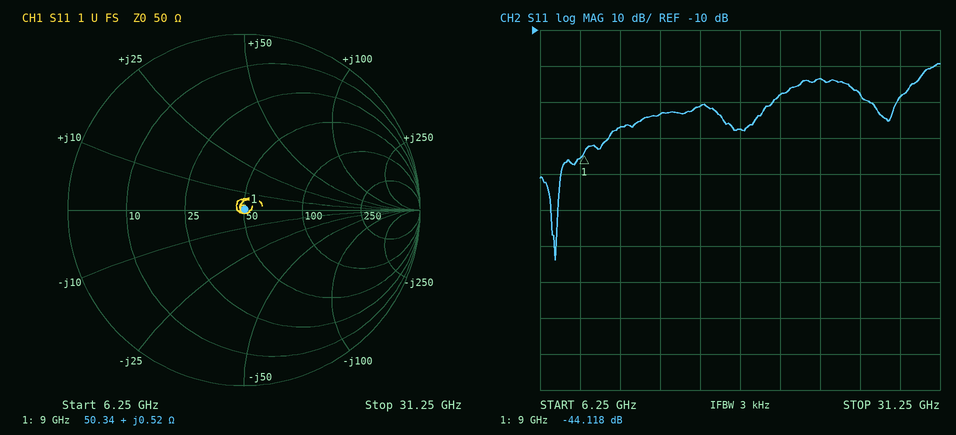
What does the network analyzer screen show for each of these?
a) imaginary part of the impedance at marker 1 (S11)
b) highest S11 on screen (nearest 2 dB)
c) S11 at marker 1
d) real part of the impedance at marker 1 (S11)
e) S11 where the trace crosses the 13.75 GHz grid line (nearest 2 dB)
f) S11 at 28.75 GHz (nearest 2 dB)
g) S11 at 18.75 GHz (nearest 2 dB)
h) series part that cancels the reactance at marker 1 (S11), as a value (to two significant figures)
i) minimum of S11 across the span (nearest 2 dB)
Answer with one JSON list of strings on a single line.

["+0.52 Ω", "-20 dB", "-44.118 dB", "50.34 Ω", "-34 dB", "-28 dB", "-38 dB", "34 pF", "-74 dB"]
